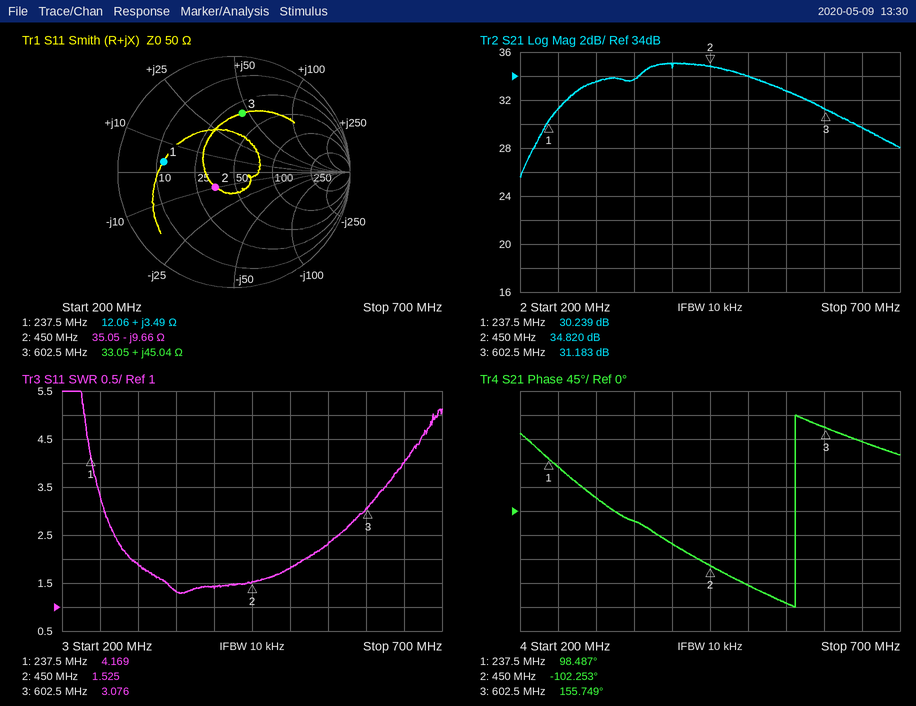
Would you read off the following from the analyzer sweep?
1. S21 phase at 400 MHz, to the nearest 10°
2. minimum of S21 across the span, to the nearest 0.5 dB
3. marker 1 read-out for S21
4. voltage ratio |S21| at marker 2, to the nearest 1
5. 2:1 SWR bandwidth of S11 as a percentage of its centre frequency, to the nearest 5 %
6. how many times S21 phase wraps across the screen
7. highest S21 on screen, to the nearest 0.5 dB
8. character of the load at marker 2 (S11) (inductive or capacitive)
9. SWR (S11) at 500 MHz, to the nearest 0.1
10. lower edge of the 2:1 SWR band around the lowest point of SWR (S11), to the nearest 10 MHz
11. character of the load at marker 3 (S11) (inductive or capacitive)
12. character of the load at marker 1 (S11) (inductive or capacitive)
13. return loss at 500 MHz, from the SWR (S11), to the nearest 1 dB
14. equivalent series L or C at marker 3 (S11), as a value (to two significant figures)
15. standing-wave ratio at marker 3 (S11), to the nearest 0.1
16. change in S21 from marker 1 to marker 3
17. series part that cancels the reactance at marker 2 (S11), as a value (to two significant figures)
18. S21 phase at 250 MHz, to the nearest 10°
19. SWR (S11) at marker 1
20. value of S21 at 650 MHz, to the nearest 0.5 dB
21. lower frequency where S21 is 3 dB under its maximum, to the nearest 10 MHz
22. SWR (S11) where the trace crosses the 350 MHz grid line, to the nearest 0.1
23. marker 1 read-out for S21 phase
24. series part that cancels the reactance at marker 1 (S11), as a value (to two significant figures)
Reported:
-60°
25.5 dB
30.239 dB
55
55 %
1
35.0 dB
capacitive
1.8
290 MHz
inductive
inductive
11 dB
12 nH
3.1
0.944 dB
3.4 nH
80°
4.169
29.5 dB
260 MHz
1.3
98.487°
190 pF
